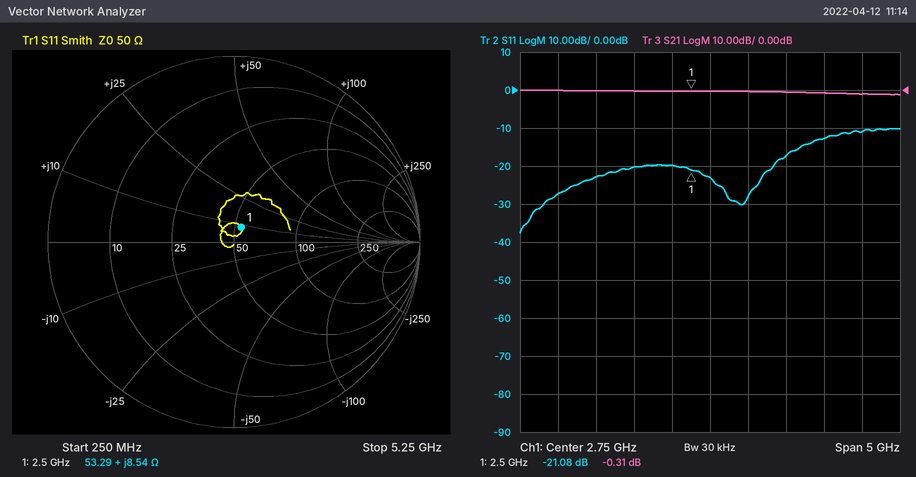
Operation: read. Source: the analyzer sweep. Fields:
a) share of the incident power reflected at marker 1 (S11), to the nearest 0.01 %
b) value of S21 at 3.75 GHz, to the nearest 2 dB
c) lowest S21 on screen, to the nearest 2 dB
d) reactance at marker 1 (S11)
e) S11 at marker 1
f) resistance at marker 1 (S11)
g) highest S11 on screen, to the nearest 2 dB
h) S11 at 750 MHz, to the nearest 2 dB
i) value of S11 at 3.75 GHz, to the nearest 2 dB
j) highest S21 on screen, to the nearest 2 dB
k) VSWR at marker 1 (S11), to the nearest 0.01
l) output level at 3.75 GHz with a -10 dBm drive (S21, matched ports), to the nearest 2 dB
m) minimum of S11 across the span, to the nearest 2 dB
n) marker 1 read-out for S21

0.78 %
0 dB
-2 dB
+8.54 Ω
-21.08 dB
53.29 Ω
-10 dB
-28 dB
-18 dB
0 dB
1.19
-10 dBm
-38 dB
-0.31 dB
